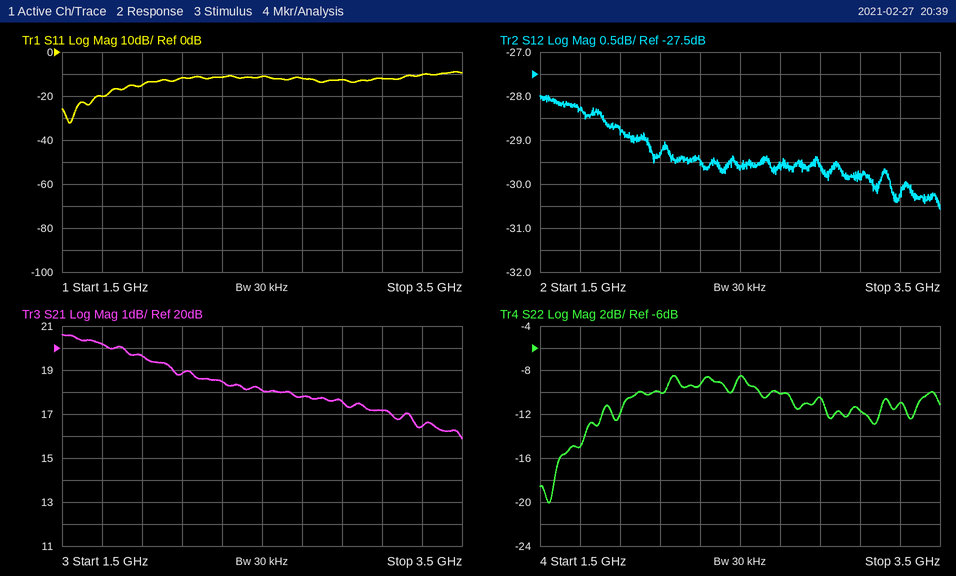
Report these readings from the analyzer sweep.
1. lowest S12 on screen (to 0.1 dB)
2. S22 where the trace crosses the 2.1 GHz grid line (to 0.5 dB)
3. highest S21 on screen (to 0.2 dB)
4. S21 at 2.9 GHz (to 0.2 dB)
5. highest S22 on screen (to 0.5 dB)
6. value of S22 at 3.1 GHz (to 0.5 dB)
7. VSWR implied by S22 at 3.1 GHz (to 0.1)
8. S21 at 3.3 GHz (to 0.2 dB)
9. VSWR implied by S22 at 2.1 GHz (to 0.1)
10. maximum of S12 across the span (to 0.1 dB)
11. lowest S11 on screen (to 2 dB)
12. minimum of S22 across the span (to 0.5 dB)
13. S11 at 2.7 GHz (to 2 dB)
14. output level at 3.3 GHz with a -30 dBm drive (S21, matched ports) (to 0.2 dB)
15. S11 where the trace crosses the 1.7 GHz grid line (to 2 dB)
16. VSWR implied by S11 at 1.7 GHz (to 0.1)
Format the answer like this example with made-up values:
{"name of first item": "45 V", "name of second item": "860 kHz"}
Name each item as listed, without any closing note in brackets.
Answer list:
{"lowest S12 on screen": "-30.6 dB", "S22 where the trace crosses the 2.1 GHz grid line": "-10.0 dB", "highest S21 on screen": "20.6 dB", "S21 at 2.9 GHz": "17.6 dB", "highest S22 on screen": "-8.5 dB", "value of S22 at 3.1 GHz": "-11.5 dB", "VSWR implied by S22 at 3.1 GHz": "1.7", "S21 at 3.3 GHz": "16.4 dB", "VSWR implied by S22 at 2.1 GHz": "1.9", "maximum of S12 across the span": "-28.0 dB", "lowest S11 on screen": "-32 dB", "minimum of S22 across the span": "-20.0 dB", "S11 at 2.7 GHz": "-12 dB", "output level at 3.3 GHz with a -30 dBm drive (S21, matched ports)": "-13.6 dBm", "S11 where the trace crosses the 1.7 GHz grid line": "-20 dB", "VSWR implied by S11 at 1.7 GHz": "1.2"}
